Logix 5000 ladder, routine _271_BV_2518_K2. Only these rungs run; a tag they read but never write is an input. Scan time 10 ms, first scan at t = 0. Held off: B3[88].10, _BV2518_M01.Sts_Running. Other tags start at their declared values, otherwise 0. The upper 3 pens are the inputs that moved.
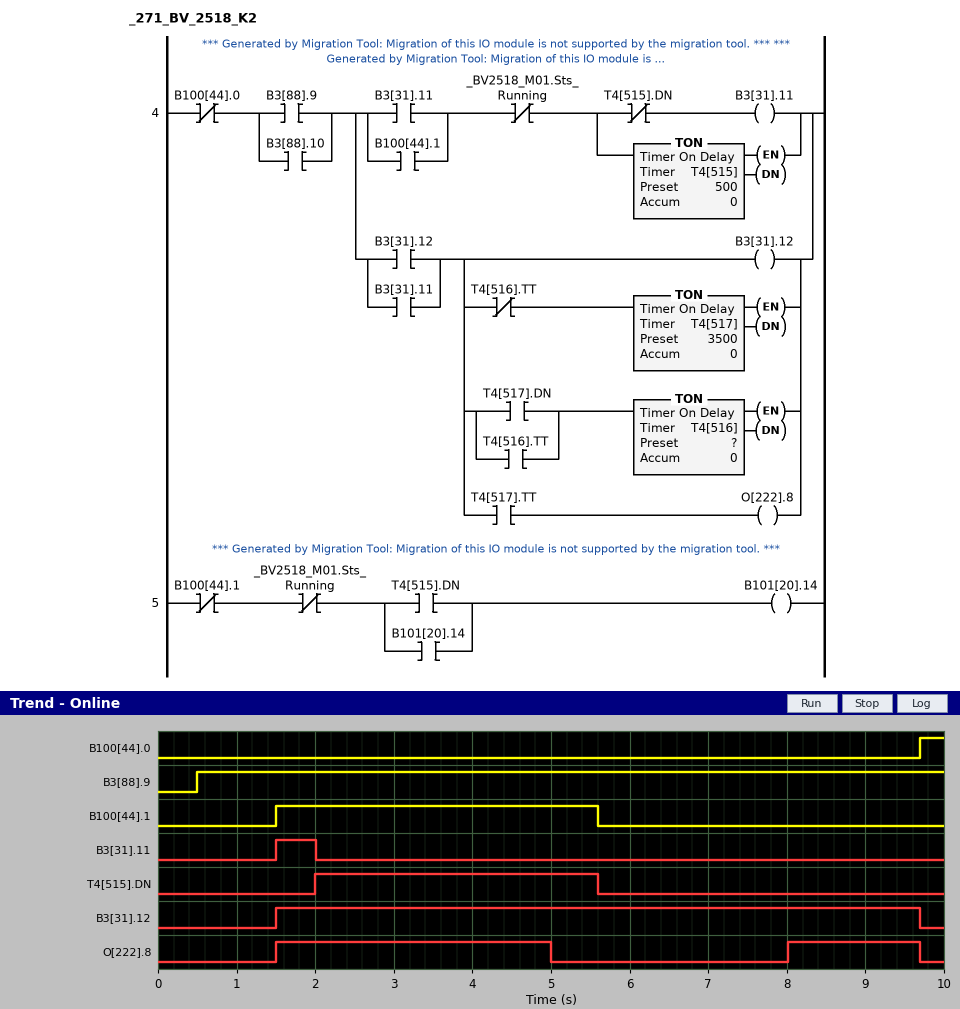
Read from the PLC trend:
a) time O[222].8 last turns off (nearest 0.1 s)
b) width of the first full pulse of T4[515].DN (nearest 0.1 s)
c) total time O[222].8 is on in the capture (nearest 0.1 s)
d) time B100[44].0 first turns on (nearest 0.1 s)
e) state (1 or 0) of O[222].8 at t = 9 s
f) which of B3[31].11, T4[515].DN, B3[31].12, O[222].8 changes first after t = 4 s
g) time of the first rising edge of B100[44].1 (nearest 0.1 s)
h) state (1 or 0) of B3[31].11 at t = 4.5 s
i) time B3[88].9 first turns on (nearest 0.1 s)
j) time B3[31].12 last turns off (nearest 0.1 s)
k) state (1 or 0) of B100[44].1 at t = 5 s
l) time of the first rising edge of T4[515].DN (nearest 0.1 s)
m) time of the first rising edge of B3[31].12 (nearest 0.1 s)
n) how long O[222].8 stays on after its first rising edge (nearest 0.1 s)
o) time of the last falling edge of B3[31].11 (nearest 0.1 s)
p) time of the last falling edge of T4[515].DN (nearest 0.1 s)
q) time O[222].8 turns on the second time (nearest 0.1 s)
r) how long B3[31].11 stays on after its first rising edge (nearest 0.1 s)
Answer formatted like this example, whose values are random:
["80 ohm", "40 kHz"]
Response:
["9.7 s", "3.6 s", "5.2 s", "9.7 s", "1", "O[222].8", "1.5 s", "0", "0.5 s", "9.7 s", "1", "2.0 s", "1.5 s", "3.5 s", "2.0 s", "5.6 s", "8.0 s", "0.5 s"]
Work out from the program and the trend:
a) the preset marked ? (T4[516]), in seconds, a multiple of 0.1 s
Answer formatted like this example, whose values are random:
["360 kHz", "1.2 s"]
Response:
["3.0 s"]
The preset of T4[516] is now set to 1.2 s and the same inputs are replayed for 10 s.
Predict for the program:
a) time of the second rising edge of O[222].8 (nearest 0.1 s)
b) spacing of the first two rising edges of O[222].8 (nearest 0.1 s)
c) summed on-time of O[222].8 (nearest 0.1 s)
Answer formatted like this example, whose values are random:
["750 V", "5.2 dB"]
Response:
["6.2 s", "4.7 s", "7.0 s"]
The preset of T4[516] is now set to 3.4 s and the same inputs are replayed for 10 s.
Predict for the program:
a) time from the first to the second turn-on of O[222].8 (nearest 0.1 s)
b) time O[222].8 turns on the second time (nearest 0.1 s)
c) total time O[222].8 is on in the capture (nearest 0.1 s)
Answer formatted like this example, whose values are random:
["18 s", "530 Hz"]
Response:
["6.9 s", "8.4 s", "4.8 s"]
